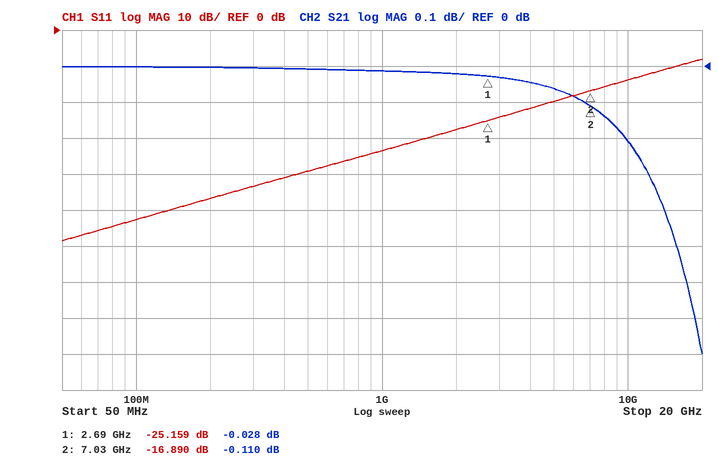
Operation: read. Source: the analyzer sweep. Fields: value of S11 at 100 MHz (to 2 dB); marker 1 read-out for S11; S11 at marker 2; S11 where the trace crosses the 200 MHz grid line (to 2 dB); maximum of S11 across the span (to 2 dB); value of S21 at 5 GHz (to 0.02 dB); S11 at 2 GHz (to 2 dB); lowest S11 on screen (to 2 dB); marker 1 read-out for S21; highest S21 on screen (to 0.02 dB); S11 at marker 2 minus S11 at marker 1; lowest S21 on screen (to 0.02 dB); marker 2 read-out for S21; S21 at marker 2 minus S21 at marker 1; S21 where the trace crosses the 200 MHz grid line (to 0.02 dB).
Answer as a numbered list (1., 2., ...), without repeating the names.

1. -52 dB
2. -25.159 dB
3. -16.890 dB
4. -46 dB
5. -8 dB
6. -0.06 dB
7. -28 dB
8. -58 dB
9. -0.028 dB
10. 0.00 dB
11. 8.269 dB
12. -0.80 dB
13. -0.110 dB
14. -0.082 dB
15. 0.00 dB
